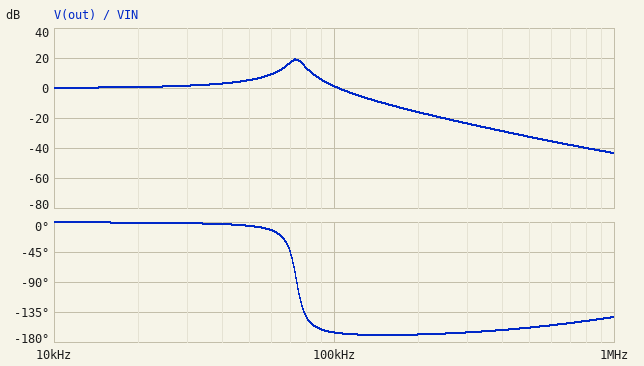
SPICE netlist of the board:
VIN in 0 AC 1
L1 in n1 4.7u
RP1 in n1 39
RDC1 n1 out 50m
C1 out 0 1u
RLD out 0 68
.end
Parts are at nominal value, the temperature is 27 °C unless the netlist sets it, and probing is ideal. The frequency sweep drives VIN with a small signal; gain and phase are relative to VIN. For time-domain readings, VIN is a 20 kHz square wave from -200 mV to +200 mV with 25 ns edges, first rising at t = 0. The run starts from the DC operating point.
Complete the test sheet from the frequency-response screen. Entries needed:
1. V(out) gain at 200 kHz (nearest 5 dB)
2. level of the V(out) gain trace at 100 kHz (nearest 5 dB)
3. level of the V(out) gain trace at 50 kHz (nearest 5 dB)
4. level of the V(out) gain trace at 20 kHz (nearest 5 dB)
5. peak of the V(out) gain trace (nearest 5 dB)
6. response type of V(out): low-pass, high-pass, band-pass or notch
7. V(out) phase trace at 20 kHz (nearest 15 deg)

-15 dB
0 dB
5 dB
0 dB
20 dB
low-pass
0 deg
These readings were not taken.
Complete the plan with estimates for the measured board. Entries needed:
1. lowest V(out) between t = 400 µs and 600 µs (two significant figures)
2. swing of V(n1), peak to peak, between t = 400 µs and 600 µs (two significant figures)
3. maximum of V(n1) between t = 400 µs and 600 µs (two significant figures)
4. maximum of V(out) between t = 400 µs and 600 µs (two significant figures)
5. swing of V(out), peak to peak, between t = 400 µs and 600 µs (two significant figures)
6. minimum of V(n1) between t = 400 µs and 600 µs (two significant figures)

-460 mV
910 mV
460 mV
460 mV
910 mV
-460 mV
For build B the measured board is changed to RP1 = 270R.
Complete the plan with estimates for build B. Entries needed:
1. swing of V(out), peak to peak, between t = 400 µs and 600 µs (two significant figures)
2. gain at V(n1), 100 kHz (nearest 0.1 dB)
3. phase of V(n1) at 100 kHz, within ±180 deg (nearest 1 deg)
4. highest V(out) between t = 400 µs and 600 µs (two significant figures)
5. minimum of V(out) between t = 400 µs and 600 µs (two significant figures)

900 mV
1.3 dB
-172 deg
450 mV
-450 mV
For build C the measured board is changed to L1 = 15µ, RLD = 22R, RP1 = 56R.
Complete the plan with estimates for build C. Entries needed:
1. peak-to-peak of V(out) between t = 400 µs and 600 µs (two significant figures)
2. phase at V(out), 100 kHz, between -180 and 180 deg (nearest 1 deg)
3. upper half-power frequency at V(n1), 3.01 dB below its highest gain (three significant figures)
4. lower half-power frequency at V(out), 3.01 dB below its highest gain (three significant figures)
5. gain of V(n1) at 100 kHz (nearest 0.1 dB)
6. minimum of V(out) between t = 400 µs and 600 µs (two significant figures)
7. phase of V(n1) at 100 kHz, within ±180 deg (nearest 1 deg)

770 mV
-163 deg
45.5 kHz
34.7 kHz
-13.8 dB
-380 mV
-161 deg
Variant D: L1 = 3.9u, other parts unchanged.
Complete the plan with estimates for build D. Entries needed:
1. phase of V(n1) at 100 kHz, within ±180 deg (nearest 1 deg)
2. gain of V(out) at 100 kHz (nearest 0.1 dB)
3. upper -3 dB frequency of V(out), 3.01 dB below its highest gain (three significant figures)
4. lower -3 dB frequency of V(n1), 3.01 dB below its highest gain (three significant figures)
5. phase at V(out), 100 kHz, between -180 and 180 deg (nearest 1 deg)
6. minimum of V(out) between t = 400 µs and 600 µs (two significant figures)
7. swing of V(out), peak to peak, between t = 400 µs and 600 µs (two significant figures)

-161 deg
5.1 dB
84.5 kHz
76.0 kHz
-163 deg
-420 mV
850 mV
